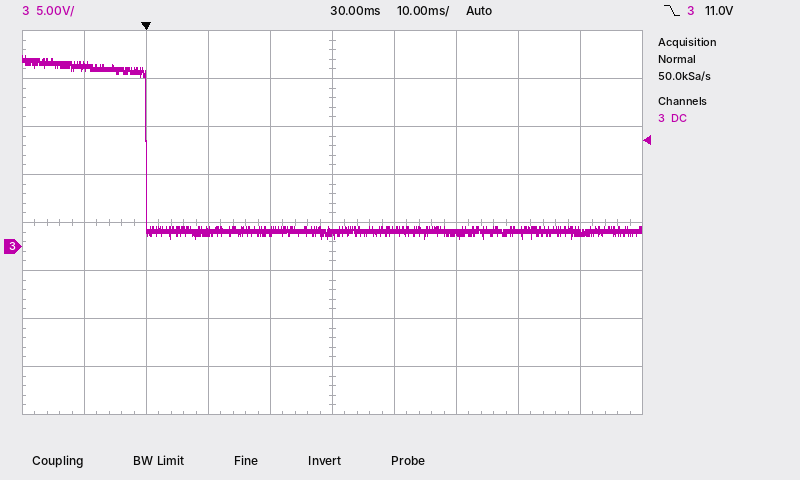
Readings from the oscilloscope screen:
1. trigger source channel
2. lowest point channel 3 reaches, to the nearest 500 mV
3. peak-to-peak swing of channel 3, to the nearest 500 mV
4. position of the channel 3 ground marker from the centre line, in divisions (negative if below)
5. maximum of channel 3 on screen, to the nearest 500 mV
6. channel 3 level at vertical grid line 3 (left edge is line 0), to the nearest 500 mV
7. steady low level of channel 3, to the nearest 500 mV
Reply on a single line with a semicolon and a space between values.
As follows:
channel 3; 1.0 V; 19.0 V; -0.5 div; 20.0 V; 1.5 V; 1.5 V
